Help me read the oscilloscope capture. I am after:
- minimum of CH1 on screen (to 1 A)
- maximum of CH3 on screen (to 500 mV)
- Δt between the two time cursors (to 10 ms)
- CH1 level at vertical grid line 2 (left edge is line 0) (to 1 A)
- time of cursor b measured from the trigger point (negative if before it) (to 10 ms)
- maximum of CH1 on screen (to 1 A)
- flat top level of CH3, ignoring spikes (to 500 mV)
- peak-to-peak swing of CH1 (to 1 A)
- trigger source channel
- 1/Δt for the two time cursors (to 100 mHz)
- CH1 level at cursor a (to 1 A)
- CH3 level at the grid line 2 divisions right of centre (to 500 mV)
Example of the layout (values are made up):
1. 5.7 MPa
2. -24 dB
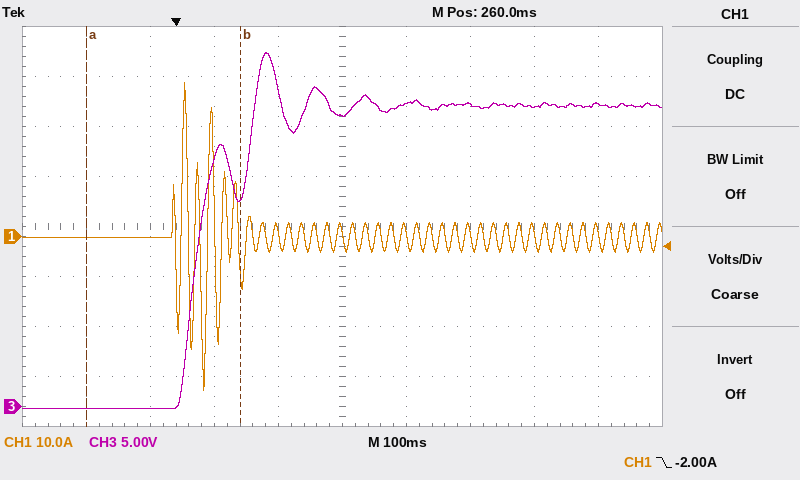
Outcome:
1. -31 A
2. 35.5 V
3. 240 ms
4. 0 A
5. +100 ms
6. 31 A
7. 30.0 V
8. 62 A
9. CH1
10. 4.2 Hz
11. 0 A
12. 30.0 V
